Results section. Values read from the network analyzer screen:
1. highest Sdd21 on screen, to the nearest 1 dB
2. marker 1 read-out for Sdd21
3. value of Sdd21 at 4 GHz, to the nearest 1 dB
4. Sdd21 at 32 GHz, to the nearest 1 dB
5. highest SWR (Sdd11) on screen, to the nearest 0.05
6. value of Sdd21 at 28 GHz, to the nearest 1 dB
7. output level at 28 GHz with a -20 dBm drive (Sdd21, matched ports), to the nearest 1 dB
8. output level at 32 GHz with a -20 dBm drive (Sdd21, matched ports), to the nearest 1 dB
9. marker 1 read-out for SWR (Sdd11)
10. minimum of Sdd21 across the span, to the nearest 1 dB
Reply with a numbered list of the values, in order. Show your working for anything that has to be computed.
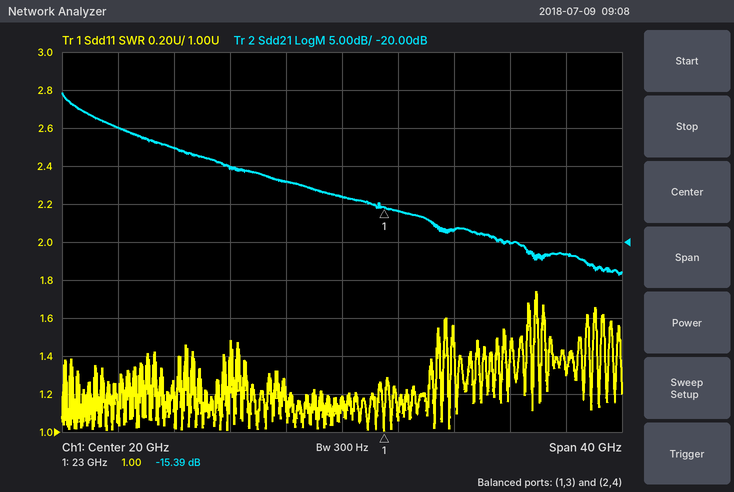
1. 0 dB
2. -15.39 dB
3. -5 dB
4. -20 dB
5. 1.75
6. -18 dB
7. -20 dBm + (-18 dB) = -38 dBm
8. -20 dBm + (-20 dB) = -40 dBm
9. 1.00
10. -24 dB
